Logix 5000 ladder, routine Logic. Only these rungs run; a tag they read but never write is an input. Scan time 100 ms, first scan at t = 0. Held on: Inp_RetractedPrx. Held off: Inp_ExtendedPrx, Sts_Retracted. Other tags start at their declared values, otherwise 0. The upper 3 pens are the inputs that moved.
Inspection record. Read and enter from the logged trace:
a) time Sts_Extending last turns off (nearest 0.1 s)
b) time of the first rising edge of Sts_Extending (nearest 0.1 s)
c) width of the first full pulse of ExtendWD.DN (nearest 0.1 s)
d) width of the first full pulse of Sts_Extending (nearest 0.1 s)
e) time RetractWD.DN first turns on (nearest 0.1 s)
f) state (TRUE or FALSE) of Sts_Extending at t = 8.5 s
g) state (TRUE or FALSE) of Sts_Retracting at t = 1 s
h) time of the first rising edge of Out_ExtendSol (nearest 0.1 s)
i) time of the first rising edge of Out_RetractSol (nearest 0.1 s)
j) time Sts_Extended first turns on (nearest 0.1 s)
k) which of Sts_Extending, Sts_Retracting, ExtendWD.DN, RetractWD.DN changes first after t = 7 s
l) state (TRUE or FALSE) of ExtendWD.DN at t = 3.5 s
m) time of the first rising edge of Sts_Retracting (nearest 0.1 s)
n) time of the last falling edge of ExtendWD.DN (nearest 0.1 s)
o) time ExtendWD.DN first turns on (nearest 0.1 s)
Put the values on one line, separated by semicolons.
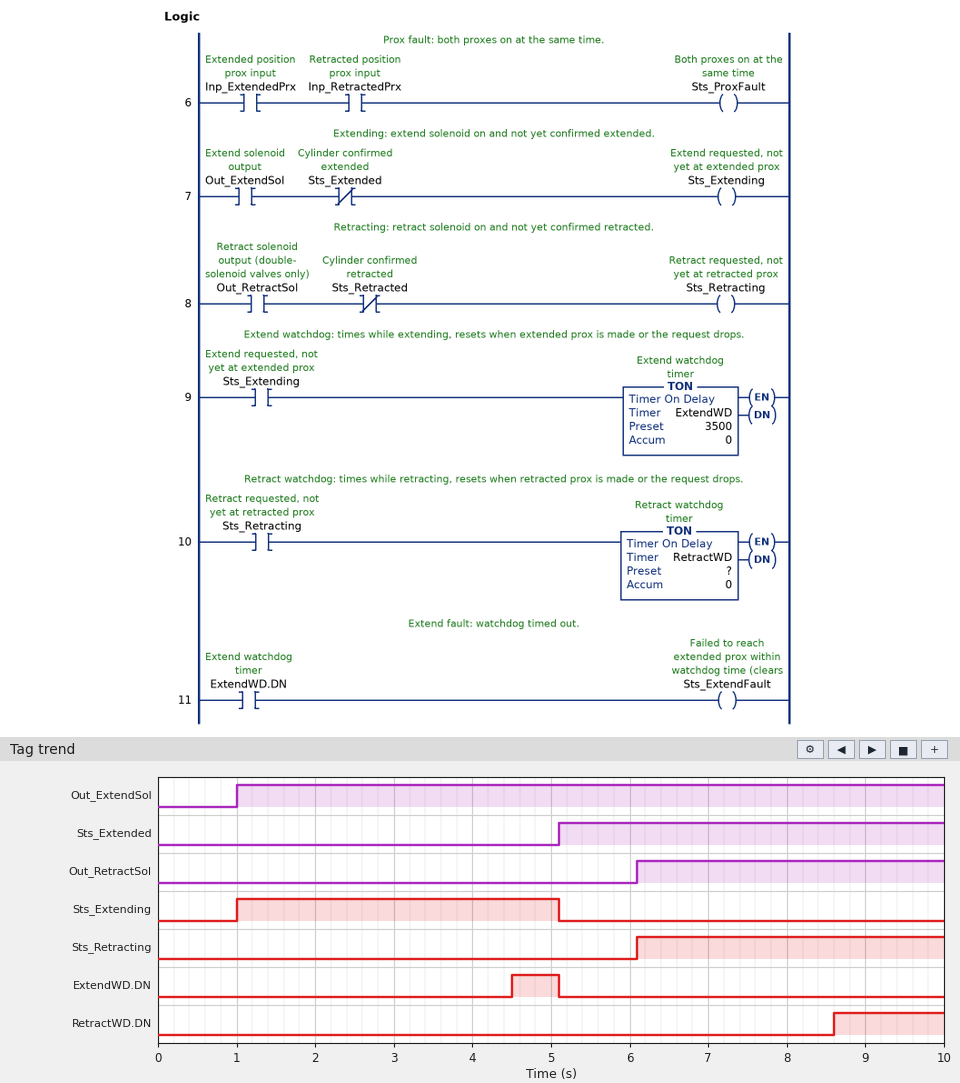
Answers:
5.1 s; 1.0 s; 0.6 s; 4.1 s; 8.6 s; FALSE; FALSE; 1.0 s; 6.1 s; 5.1 s; RetractWD.DN; FALSE; 6.1 s; 5.1 s; 4.5 s
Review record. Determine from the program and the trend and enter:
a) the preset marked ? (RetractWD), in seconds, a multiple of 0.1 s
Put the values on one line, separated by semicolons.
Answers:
2.5 s
